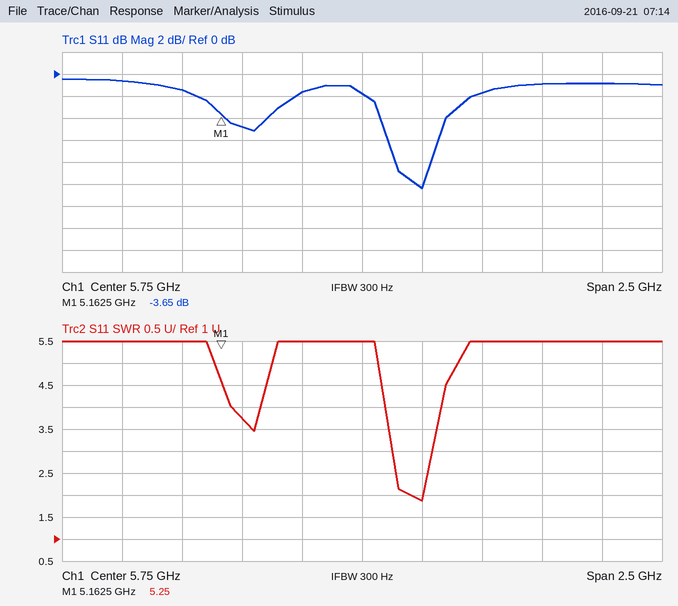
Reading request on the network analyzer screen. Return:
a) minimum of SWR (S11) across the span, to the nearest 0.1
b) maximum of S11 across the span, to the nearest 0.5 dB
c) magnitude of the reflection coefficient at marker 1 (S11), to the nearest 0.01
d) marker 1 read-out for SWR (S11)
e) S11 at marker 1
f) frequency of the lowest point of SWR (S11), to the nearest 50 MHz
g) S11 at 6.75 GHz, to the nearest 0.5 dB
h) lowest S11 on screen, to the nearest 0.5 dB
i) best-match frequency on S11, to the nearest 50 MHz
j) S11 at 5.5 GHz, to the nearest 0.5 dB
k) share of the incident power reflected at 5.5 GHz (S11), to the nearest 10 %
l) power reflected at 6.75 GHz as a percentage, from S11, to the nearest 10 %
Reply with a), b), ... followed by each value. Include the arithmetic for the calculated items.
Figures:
a) 1.9
b) -0.5 dB
c) 10^(-3.65/20) ≈ 0.66
d) 5.25
e) -3.65 dB
f) 6.00 GHz
g) -1.0 dB
h) -10.5 dB
i) 6.00 GHz
j) -1.5 dB
k) 10^(-1.5/10) ≈ 70.8 %, so 70 % to the nearest 10 %
l) 10^(-1/10) ≈ 79.4 %, so 80 % to the nearest 10 %
